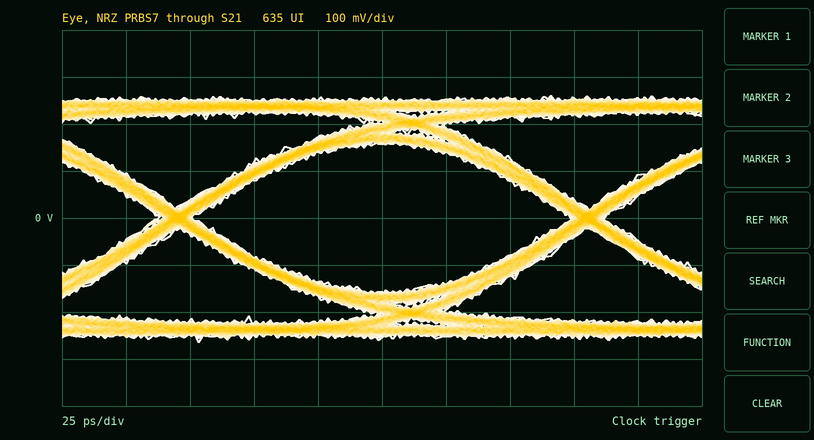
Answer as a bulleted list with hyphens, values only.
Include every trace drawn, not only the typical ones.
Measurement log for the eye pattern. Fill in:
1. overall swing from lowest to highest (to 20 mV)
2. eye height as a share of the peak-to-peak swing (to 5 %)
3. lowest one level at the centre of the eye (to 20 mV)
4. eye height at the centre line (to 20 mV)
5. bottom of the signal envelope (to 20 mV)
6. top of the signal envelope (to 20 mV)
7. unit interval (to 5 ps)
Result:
- 520 mV
- 60 %
- 160 mV
- 320 mV
- -260 mV
- 260 mV
- 160 ps
